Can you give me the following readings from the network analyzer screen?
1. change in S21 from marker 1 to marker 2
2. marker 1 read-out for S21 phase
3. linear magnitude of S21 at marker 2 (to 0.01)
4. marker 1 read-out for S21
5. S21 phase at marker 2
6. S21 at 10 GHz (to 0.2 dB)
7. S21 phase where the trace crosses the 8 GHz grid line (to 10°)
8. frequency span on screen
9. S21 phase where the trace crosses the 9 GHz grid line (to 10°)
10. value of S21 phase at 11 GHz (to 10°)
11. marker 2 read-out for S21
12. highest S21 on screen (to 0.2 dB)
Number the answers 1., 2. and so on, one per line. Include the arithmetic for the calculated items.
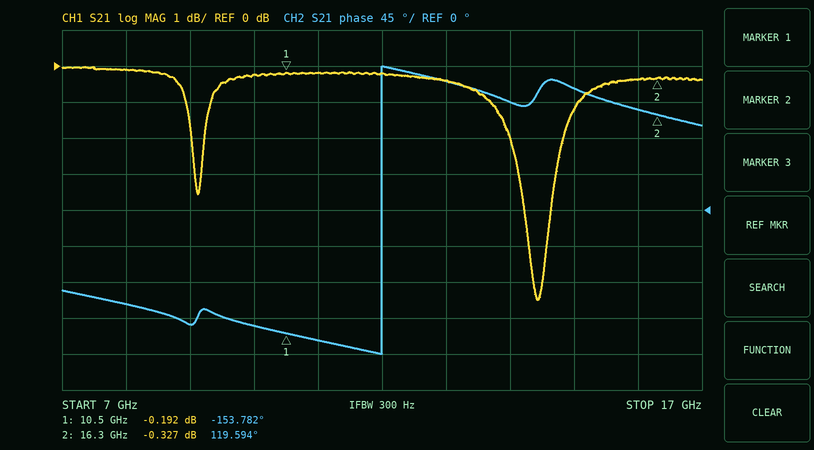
1. -0.327 − (-0.192) = -0.135 dB
2. -153.782°
3. 10^(-0.327/20) ≈ 0.96
4. -0.192 dB
5. 119.594°
6. -0.2 dB
7. -120°
8. 10 GHz
9. -140°
10. -160°
11. -0.327 dB
12. 0.0 dB
